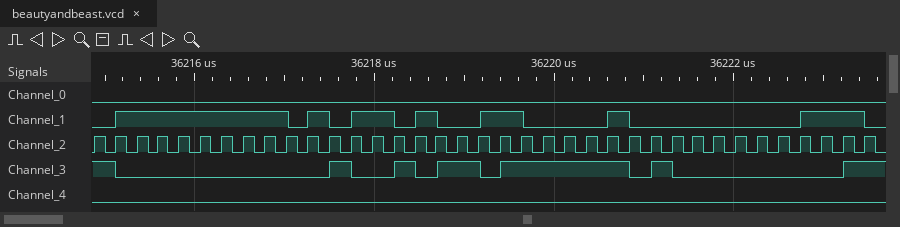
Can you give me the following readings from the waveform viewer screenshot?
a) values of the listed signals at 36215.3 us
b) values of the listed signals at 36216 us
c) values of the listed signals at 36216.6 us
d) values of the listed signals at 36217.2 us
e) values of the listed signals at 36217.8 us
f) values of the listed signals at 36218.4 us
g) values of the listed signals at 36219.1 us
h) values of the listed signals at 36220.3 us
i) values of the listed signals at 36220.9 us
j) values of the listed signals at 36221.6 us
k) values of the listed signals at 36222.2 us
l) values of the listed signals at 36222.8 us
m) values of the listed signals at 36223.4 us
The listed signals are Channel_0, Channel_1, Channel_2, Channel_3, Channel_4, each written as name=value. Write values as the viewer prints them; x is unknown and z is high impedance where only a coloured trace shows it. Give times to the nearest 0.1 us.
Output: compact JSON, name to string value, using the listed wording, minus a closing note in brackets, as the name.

{"values of the listed signals at 36215.3 us": "Channel_0=0, Channel_1=1, Channel_2=0, Channel_3=0, Channel_4=0", "values of the listed signals at 36216 us": "Channel_0=0, Channel_1=1, Channel_2=0, Channel_3=0, Channel_4=0", "values of the listed signals at 36216.6 us": "Channel_0=0, Channel_1=1, Channel_2=1, Channel_3=0, Channel_4=0", "values of the listed signals at 36217.2 us": "Channel_0=0, Channel_1=0, Channel_2=0, Channel_3=0, Channel_4=0", "values of the listed signals at 36217.8 us": "Channel_0=0, Channel_1=1, Channel_2=1, Channel_3=0, Channel_4=0", "values of the listed signals at 36218.4 us": "Channel_0=0, Channel_1=0, Channel_2=0, Channel_3=1, Channel_4=0", "values of the listed signals at 36219.1 us": "Channel_0=0, Channel_1=0, Channel_2=0, Channel_3=1, Channel_4=0", "values of the listed signals at 36220.3 us": "Channel_0=0, Channel_1=0, Channel_2=0, Channel_3=1, Channel_4=0", "values of the listed signals at 36220.9 us": "Channel_0=0, Channel_1=0, Channel_2=1, Channel_3=0, Channel_4=0", "values of the listed signals at 36221.6 us": "Channel_0=0, Channel_1=0, Channel_2=1, Channel_3=0, Channel_4=0", "values of the listed signals at 36222.2 us": "Channel_0=0, Channel_1=0, Channel_2=0, Channel_3=0, Channel_4=0", "values of the listed signals at 36222.8 us": "Channel_0=0, Channel_1=1, Channel_2=1, Channel_3=0, Channel_4=0", "values of the listed signals at 36223.4 us": "Channel_0=0, Channel_1=1, Channel_2=0, Channel_3=1, Channel_4=0"}
